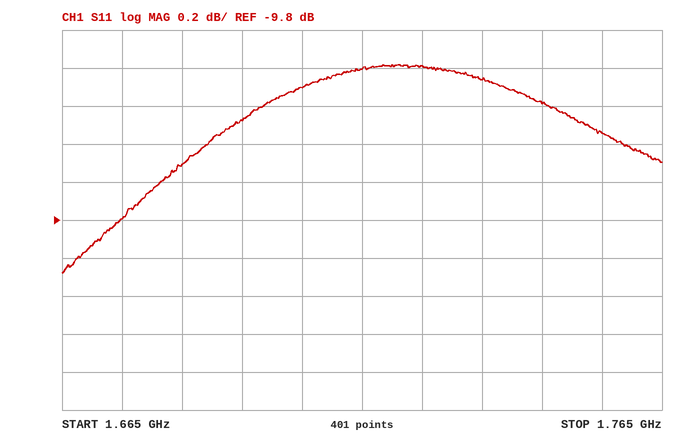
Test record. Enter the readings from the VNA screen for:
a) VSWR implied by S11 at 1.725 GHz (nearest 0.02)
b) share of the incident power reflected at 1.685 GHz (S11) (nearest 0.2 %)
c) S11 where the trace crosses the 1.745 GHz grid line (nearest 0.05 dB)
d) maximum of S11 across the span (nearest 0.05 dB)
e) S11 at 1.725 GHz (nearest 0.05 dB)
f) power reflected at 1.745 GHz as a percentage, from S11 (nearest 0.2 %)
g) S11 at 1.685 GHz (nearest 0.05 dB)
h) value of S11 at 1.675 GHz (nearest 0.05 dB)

2.10
11.2 %
-9.20 dB
-9.00 dB
-9.00 dB
12.0 %
-9.50 dB
-9.80 dB
